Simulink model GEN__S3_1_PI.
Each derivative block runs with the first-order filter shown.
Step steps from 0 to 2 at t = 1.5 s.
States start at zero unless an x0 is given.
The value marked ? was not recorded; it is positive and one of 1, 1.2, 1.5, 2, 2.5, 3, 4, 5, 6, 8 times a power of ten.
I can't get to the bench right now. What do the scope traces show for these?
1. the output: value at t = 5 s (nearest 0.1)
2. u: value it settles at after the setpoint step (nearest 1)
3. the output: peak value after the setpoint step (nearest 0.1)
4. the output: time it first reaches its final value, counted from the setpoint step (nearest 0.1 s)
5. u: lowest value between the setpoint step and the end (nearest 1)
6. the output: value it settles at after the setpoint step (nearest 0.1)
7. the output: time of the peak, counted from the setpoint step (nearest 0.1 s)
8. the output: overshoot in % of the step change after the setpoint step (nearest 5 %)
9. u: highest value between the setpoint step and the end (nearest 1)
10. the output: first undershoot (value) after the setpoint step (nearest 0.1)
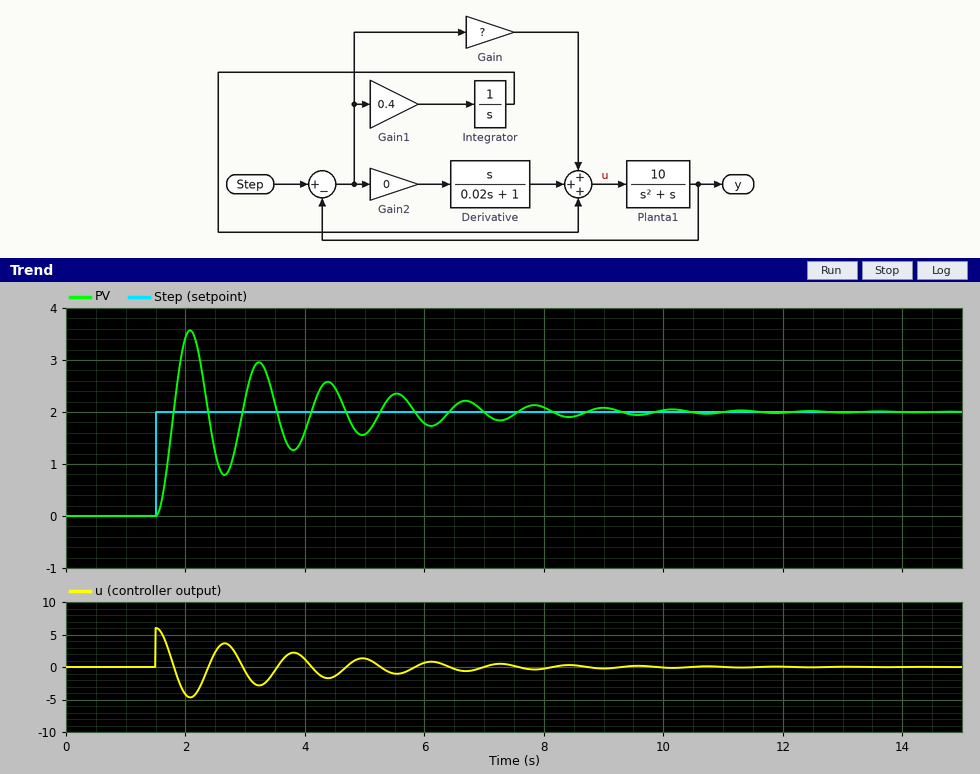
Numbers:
1.6
0
3.6
0.3 s
-5
2.0
0.6 s
80 %
6
0.8
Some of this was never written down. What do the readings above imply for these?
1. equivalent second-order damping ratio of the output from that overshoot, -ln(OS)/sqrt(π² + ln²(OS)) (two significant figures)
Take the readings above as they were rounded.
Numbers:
0.071
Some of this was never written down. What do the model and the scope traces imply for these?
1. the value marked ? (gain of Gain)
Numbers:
3
